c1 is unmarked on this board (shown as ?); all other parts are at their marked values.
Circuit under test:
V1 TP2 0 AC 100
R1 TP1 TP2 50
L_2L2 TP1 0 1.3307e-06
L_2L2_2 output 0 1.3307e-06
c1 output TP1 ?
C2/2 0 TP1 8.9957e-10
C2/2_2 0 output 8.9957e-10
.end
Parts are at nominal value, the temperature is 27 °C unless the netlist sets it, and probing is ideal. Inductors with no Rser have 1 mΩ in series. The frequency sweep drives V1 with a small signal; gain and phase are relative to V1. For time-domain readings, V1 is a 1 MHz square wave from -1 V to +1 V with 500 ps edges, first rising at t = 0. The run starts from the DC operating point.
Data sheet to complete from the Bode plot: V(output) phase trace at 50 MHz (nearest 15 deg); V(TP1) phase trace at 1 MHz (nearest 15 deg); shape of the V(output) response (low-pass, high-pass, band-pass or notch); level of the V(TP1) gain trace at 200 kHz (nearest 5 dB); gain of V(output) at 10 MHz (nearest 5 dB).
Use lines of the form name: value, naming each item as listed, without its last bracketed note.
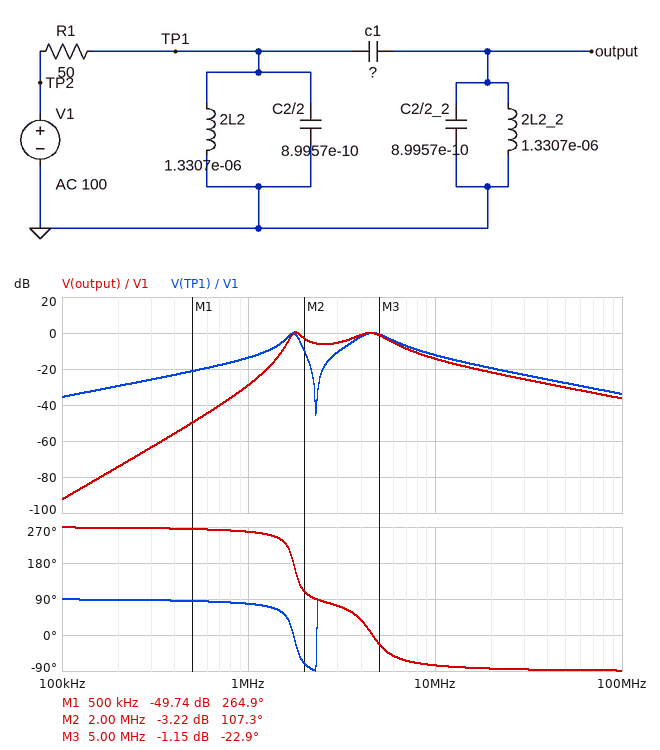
V(output) phase trace at 50 MHz: -90 deg
V(TP1) phase trace at 1 MHz: 75 deg
shape of the V(output) response: band-pass
level of the V(TP1) gain trace at 200 kHz: -30 dB
gain of V(output) at 10 MHz: -15 dB
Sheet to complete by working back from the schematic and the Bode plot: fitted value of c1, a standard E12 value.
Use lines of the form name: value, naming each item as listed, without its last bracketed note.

fitted value of c1, a standard E12 value: 2.7 nF
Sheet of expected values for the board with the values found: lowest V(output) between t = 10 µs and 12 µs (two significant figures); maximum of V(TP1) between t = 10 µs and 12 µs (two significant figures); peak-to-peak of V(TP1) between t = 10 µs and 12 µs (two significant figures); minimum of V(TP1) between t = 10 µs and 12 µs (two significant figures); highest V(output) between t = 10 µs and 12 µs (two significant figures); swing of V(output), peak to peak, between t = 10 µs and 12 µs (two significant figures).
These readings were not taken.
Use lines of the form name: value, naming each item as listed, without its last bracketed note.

lowest V(output) between t = 10 µs and 12 µs: -460 mV
maximum of V(TP1) between t = 10 µs and 12 µs: 700 mV
peak-to-peak of V(TP1) between t = 10 µs and 12 µs: 1.4 V
minimum of V(TP1) between t = 10 µs and 12 µs: -700 mV
highest V(output) between t = 10 µs and 12 µs: 460 mV
swing of V(output), peak to peak, between t = 10 µs and 12 µs: 930 mV
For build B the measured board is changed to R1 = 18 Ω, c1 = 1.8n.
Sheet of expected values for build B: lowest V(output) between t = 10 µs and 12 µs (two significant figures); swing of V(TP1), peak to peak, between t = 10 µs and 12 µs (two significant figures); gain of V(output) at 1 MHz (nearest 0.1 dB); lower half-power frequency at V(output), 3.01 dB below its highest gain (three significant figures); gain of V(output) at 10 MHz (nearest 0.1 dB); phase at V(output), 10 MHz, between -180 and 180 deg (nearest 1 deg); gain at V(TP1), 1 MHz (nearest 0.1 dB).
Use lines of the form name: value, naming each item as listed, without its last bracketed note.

lowest V(output) between t = 10 µs and 12 µs: -1.0 V
swing of V(TP1), peak to peak, between t = 10 µs and 12 µs: 2.7 V
gain of V(output) at 1 MHz: -25.5 dB
lower half-power frequency at V(output), 3.01 dB below its highest gain: 2.19 MHz
gain of V(output) at 10 MHz: -7.5 dB
phase at V(output), 10 MHz, between -180 and 180 deg: -54 deg
gain at V(TP1), 1 MHz: -6.4 dB
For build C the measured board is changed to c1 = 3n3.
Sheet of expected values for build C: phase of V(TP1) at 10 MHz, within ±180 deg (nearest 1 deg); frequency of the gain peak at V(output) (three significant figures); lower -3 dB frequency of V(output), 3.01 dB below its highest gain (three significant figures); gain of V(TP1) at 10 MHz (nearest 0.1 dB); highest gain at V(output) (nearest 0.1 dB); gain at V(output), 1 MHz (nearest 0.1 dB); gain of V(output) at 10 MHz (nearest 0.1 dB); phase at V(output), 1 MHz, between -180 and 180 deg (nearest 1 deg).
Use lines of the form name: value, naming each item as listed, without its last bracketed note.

phase of V(TP1) at 10 MHz, within ±180 deg: -76 deg
frequency of the gain peak at V(output): 1.63 MHz
lower -3 dB frequency of V(output), 3.01 dB below its highest gain: 1.53 MHz
gain of V(TP1) at 10 MHz: -12.4 dB
highest gain at V(output): 0.4 dB
gain at V(output), 1 MHz: -26.2 dB
gain of V(output) at 10 MHz: -14.1 dB
phase at V(output), 1 MHz, between -180 and 180 deg: -103 deg
